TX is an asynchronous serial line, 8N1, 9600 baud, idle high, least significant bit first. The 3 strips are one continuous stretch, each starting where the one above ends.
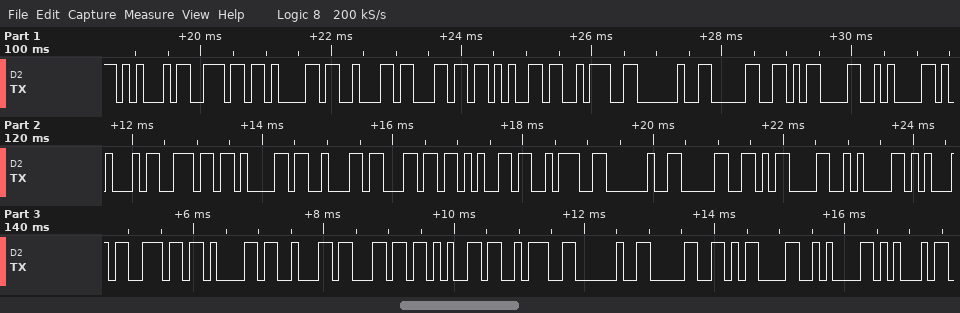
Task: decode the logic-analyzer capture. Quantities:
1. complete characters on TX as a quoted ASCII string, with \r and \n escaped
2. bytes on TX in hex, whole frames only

"Enable: 0\r\nEnable: 0\r\nEnable: 0\r\nE"
0x45 0x6E 0x61 0x62 0x6C 0x65 0x3A 0x20 0x30 0x0D 0x0A 0x45 0x6E 0x61 0x62 0x6C 0x65 0x3A 0x20 0x30 0x0D 0x0A 0x45 0x6E 0x61 0x62 0x6C 0x65 0x3A 0x20 0x30 0x0D 0x0A 0x45
